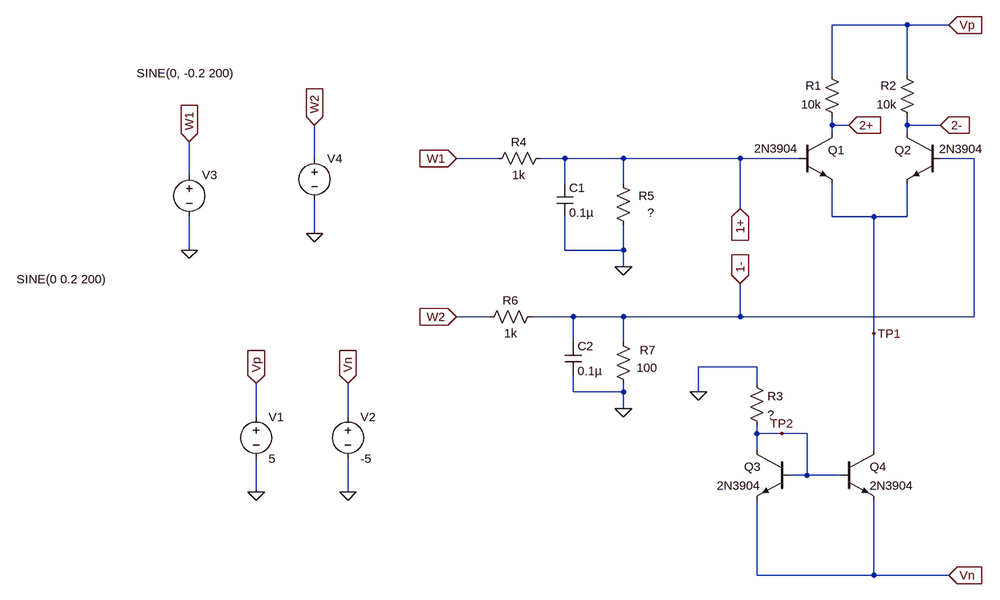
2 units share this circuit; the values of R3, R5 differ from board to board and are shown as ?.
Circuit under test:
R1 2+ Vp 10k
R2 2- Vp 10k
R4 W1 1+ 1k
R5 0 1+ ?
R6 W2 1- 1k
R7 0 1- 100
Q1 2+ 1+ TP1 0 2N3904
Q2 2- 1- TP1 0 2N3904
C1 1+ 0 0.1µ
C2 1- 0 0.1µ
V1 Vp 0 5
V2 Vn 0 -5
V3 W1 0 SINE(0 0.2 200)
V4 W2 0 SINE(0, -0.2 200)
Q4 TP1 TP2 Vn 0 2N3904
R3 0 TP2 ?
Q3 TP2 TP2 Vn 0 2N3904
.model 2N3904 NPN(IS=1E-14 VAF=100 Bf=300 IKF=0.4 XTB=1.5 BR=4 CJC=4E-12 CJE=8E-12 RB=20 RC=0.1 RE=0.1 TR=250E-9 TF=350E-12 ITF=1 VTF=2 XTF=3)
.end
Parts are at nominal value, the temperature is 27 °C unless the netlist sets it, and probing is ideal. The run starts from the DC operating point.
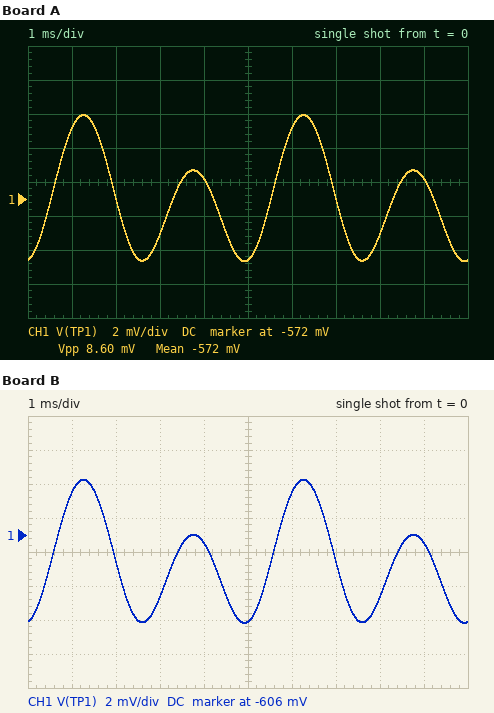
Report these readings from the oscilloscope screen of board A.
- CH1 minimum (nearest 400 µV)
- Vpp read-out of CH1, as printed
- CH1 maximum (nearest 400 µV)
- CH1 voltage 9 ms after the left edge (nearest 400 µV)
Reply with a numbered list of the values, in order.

1. -575.6 mV
2. 8.60 mV
3. -567.2 mV
4. -570.8 mV
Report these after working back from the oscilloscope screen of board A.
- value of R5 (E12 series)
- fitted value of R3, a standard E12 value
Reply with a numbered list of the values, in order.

1. 120 Ω
2. 47 kΩ
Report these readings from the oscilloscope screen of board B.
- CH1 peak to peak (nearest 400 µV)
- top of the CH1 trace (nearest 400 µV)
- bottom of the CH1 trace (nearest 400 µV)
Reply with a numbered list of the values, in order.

1. 8.4 mV
2. -602.8 mV
3. -611.2 mV
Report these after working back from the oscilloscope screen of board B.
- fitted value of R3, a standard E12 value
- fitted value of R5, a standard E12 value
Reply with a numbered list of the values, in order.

1. 12 kΩ
2. 120 Ω
